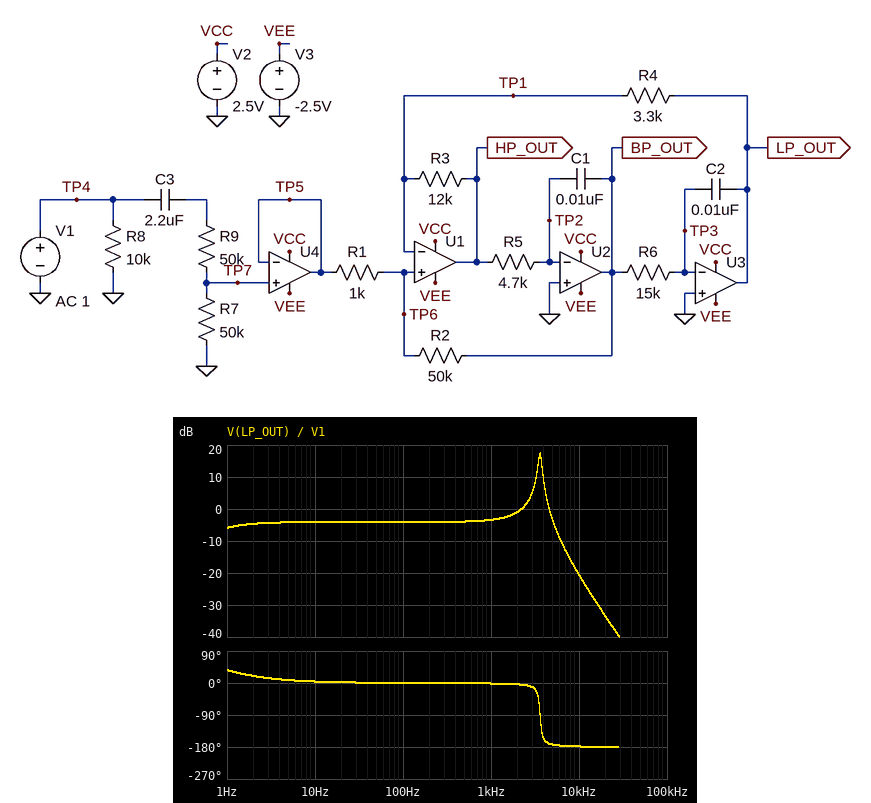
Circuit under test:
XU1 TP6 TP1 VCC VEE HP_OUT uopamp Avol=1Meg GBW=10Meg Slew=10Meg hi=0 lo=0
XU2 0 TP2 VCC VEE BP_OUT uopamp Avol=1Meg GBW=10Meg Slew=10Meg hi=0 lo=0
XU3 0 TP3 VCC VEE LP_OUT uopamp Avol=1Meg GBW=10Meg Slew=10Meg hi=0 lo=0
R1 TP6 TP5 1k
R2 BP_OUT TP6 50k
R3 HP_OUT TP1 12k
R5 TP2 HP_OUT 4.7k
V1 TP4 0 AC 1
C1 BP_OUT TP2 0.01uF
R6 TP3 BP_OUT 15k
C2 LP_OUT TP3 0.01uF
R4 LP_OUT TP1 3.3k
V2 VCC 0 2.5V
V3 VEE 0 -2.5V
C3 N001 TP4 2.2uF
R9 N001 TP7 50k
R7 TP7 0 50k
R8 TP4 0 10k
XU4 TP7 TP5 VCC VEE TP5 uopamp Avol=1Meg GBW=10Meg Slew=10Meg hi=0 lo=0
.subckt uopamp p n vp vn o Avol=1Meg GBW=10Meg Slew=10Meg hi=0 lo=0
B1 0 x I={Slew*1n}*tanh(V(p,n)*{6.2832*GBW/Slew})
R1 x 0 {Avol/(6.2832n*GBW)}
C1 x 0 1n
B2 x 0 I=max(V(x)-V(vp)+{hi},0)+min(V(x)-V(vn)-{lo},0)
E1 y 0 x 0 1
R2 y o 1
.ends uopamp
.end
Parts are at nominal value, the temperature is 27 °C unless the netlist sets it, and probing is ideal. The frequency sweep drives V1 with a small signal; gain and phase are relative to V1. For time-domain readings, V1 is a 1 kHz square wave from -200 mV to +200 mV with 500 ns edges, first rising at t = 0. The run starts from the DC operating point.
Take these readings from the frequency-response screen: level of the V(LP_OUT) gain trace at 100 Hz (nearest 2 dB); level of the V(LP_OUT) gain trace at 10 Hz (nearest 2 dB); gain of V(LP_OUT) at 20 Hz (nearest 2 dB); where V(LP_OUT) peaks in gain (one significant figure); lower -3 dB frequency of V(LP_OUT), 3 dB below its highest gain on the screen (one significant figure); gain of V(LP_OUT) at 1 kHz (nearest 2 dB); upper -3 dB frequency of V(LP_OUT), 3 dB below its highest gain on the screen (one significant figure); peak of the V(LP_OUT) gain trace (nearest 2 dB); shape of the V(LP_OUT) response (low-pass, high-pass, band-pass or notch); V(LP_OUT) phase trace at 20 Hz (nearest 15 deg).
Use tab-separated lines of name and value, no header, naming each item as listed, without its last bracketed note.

level of the V(LP_OUT) gain trace at 100 Hz	-4 dB
level of the V(LP_OUT) gain trace at 10 Hz	-4 dB
gain of V(LP_OUT) at 20 Hz	-4 dB
where V(LP_OUT) peaks in gain	4 kHz
lower -3 dB frequency of V(LP_OUT), 3 dB below its highest gain on the screen	3 kHz
gain of V(LP_OUT) at 1 kHz	-4 dB
upper -3 dB frequency of V(LP_OUT), 3 dB below its highest gain on the screen	4 kHz
peak of the V(LP_OUT) gain trace	18 dB
shape of the V(LP_OUT) response	band-pass
V(LP_OUT) phase trace at 20 Hz	0 deg
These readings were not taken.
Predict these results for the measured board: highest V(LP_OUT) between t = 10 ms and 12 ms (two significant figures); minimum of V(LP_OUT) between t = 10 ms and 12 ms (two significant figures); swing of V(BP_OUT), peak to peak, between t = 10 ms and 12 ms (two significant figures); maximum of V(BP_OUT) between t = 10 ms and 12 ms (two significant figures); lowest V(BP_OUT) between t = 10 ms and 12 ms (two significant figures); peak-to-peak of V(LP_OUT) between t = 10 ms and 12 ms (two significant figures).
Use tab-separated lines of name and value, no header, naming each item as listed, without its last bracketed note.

highest V(LP_OUT) between t = 10 ms and 12 ms	410 mV
minimum of V(LP_OUT) between t = 10 ms and 12 ms	-170 mV
swing of V(BP_OUT), peak to peak, between t = 10 ms and 12 ms	1.2 V
maximum of V(BP_OUT) between t = 10 ms and 12 ms	600 mV
lowest V(BP_OUT) between t = 10 ms and 12 ms	-600 mV
peak-to-peak of V(LP_OUT) between t = 10 ms and 12 ms	580 mV
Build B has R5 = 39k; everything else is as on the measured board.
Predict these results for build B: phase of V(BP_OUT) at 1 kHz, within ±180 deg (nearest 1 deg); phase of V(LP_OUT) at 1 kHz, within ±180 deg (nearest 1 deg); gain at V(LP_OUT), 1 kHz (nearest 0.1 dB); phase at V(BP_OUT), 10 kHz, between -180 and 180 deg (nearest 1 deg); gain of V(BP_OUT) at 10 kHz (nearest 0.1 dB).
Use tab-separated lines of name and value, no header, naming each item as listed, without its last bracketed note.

phase of V(BP_OUT) at 1 kHz, within ±180 deg	-94 deg
phase of V(LP_OUT) at 1 kHz, within ±180 deg	-4 deg
gain at V(LP_OUT), 1 kHz	4.7 dB
phase at V(BP_OUT), 10 kHz, between -180 and 180 deg	90 deg
gain of V(BP_OUT) at 10 kHz	-20.5 dB
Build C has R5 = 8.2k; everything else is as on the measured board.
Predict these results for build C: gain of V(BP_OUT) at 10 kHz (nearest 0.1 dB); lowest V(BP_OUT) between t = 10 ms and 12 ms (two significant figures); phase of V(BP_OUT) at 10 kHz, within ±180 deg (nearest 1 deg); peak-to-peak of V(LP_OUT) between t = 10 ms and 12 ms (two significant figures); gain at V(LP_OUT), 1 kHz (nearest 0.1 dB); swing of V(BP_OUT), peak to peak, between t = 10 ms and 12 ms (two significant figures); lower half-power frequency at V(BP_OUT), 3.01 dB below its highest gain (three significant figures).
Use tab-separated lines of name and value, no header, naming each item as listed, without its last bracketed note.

gain of V(BP_OUT) at 10 kHz	-6.4 dB
lowest V(BP_OUT) between t = 10 ms and 12 ms	-800 mV
phase of V(BP_OUT) at 10 kHz, within ±180 deg	91 deg
peak-to-peak of V(LP_OUT) between t = 10 ms and 12 ms	840 mV
gain at V(LP_OUT), 1 kHz	-2.8 dB
swing of V(BP_OUT), peak to peak, between t = 10 ms and 12 ms	1.6 V
lower half-power frequency at V(BP_OUT), 3.01 dB below its highest gain	2.65 kHz
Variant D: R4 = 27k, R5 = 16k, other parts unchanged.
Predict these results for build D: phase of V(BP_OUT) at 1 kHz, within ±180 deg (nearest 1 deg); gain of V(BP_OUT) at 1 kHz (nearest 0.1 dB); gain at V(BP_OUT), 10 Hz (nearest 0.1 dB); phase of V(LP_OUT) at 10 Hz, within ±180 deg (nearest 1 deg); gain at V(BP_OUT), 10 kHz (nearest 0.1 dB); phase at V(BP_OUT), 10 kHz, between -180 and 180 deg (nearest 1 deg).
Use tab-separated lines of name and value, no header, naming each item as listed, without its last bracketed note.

phase of V(BP_OUT) at 1 kHz, within ±180 deg	93 deg
gain of V(BP_OUT) at 1 kHz	2.4 dB
gain at V(BP_OUT), 10 Hz	-36.5 dB
phase of V(LP_OUT) at 10 Hz, within ±180 deg	4 deg
gain at V(BP_OUT), 10 kHz	-23.0 dB
phase at V(BP_OUT), 10 kHz, between -180 and 180 deg	90 deg
